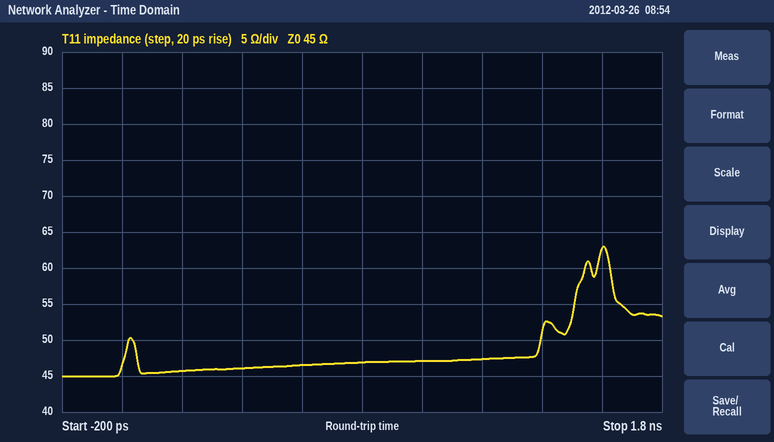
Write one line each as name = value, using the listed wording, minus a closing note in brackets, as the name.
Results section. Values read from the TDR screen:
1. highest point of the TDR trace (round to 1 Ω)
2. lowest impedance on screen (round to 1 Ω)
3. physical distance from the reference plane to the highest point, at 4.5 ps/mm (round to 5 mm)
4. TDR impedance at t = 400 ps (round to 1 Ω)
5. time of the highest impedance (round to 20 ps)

highest point of the TDR trace = 63 Ω
lowest impedance on screen = 45 Ω
physical distance from the reference plane to the highest point, at 4.5 ps/mm = 180 mm
TDR impedance at t = 400 ps = 46 Ω
time of the highest impedance = 1.60 ns
